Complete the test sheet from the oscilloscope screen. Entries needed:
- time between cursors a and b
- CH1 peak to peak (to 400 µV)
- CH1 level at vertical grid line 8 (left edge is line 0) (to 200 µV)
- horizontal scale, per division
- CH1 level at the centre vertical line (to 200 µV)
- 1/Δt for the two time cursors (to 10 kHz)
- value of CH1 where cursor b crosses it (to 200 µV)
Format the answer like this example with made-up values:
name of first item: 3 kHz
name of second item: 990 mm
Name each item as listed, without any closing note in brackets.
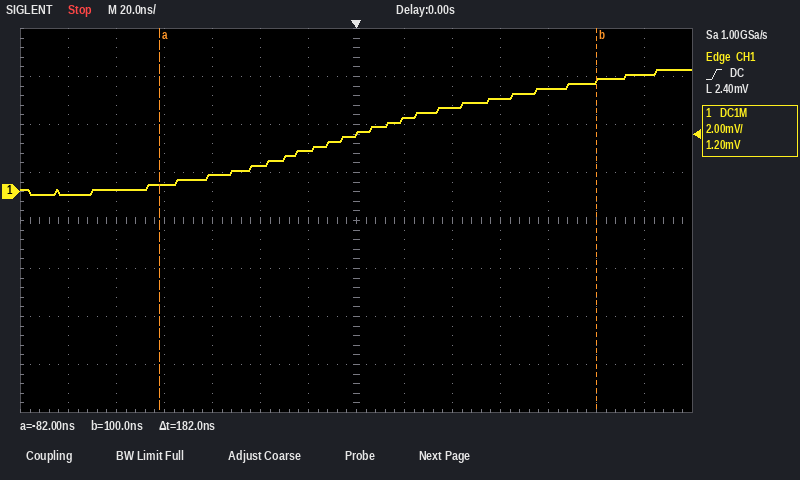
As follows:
time between cursors a and b: 182 ns
CH1 peak to peak: 5.2 mV
CH1 level at vertical grid line 8 (left edge is line 0): 3.0 mV
horizontal scale, per division: 20 ns
CH1 level at the centre vertical line: 2.4 mV
1/Δt for the two time cursors: 5.49 MHz
value of CH1 where cursor b crosses it: 4.6 mV
